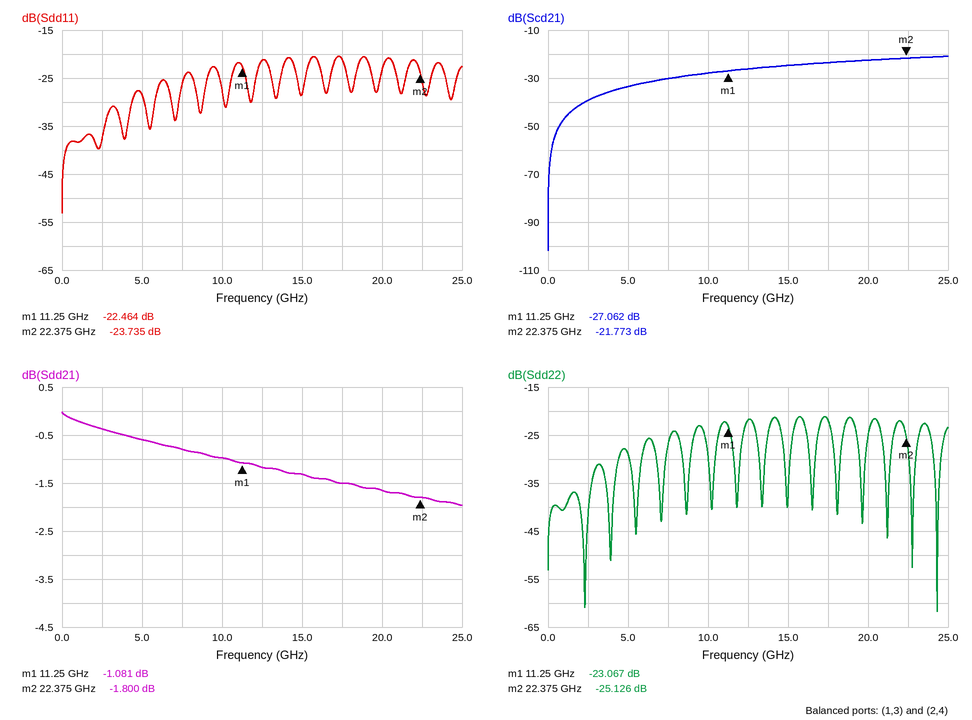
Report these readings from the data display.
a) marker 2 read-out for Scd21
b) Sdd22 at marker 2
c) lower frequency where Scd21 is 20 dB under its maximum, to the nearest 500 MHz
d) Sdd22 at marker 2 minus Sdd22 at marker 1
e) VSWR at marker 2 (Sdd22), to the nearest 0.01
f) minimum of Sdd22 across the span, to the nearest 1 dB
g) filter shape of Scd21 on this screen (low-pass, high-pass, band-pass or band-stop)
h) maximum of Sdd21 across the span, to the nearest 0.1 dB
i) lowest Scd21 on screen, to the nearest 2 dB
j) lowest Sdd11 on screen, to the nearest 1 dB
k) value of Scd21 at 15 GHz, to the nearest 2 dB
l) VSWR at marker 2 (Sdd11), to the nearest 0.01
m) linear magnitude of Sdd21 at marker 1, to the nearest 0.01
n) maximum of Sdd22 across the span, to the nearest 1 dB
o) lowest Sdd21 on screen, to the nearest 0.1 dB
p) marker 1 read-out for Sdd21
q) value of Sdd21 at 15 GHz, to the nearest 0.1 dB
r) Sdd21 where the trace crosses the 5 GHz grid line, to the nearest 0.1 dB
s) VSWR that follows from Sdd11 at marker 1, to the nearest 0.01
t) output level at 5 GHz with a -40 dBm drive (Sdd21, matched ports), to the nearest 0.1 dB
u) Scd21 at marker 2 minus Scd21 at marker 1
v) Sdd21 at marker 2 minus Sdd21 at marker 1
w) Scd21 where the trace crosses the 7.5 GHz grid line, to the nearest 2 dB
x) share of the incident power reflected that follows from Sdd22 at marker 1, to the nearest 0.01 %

-21.773 dB
-25.126 dB
2.0 GHz
-2.059 dB
1.12
-62 dB
high-pass
0.0 dB
-102 dB
-53 dB
-24 dB
1.14
0.88
-21 dB
-2.0 dB
-1.081 dB
-1.3 dB
-0.6 dB
1.16
-40.6 dBm
5.289 dB
-0.719 dB
-30 dB
0.49 %
